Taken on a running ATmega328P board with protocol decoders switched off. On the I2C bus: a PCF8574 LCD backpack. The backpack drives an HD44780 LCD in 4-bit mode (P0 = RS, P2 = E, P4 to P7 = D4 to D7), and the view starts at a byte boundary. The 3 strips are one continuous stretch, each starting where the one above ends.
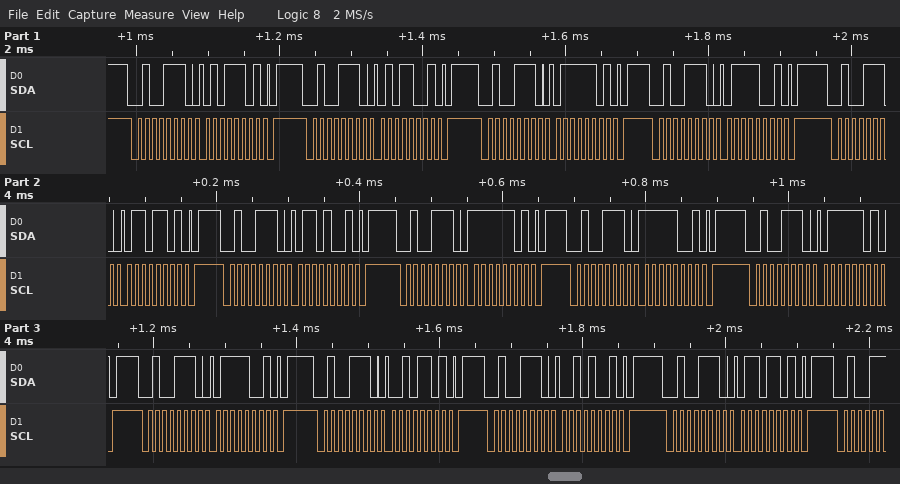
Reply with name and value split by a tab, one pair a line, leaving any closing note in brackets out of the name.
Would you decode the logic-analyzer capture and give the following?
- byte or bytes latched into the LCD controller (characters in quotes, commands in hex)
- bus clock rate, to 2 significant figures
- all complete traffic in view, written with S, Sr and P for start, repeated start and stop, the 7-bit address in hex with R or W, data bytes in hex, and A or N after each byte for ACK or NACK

byte or bytes latched into the LCD controller	'W' 'o' 'r'
bus clock rate, to 2 significant figures	100 kHz
all complete traffic in view, written with S, Sr and P for start, repeated start and stop, the 7-bit address in hex with R or W, data bytes in hex, and A or N after each byte for ACK or NACK	S 27W A 5D A P S 27W A 59 A P S 27W A 7D A P S 27W A 79 A P S 27W A 6D A P S 27W A 69 A P S 27W A FD A P S 27W A F9 A P S 27W A 7D A P S 27W A 79 A P S 27W A 2D A P S 27W A 29 A P S 27W A 6D A P
